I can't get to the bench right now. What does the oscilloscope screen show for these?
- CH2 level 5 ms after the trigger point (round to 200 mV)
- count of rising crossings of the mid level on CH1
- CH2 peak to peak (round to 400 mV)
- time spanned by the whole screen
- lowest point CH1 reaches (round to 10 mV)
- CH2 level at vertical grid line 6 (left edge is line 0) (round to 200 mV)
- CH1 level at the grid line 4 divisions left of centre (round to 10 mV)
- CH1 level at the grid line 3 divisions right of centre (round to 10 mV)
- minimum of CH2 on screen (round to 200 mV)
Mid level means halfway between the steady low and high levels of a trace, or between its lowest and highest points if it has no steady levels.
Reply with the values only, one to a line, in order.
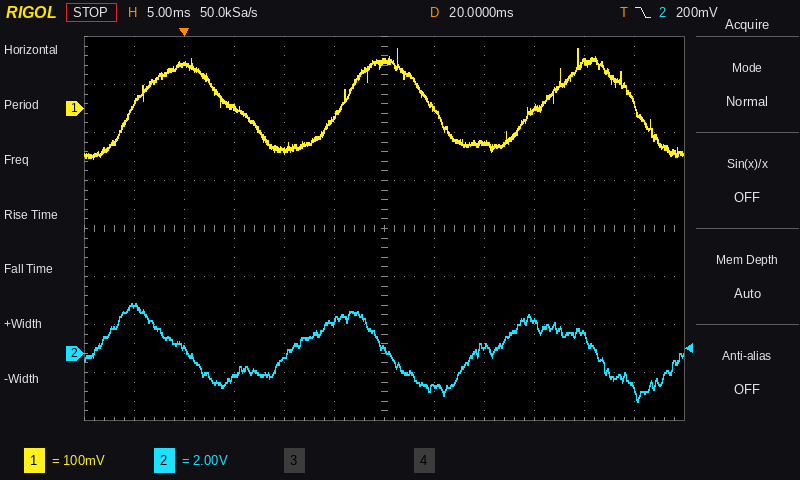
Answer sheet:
-1.0 V
3
4.0 V
60 ms
-100 mV
200 mV
90 mV
0 mV
-2.0 V
